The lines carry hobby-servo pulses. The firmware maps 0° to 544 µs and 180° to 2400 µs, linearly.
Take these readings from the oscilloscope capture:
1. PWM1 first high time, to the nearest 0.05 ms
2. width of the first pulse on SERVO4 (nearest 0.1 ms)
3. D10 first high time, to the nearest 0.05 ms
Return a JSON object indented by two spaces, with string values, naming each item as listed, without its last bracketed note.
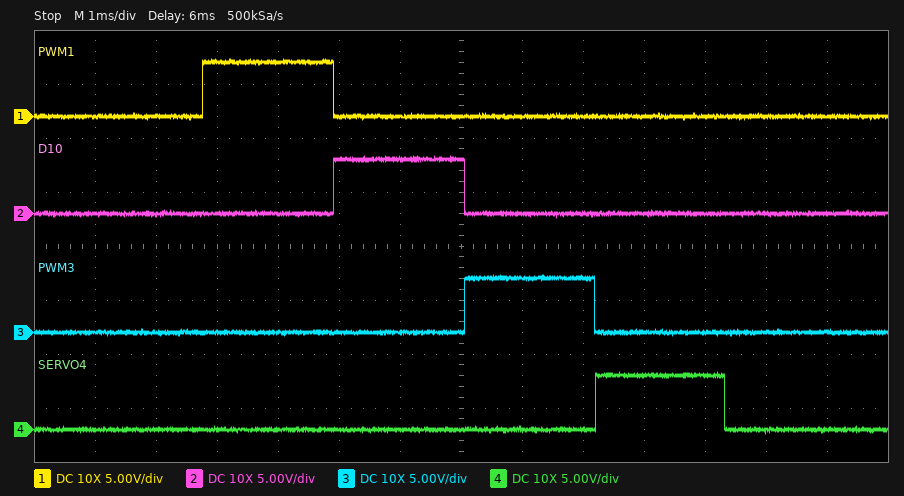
{
  "PWM1 first high time, to the nearest 0.05 ms": "2.15 ms",
  "width of the first pulse on SERVO4": "2.1 ms",
  "D10 first high time, to the nearest 0.05 ms": "2.15 ms"
}
